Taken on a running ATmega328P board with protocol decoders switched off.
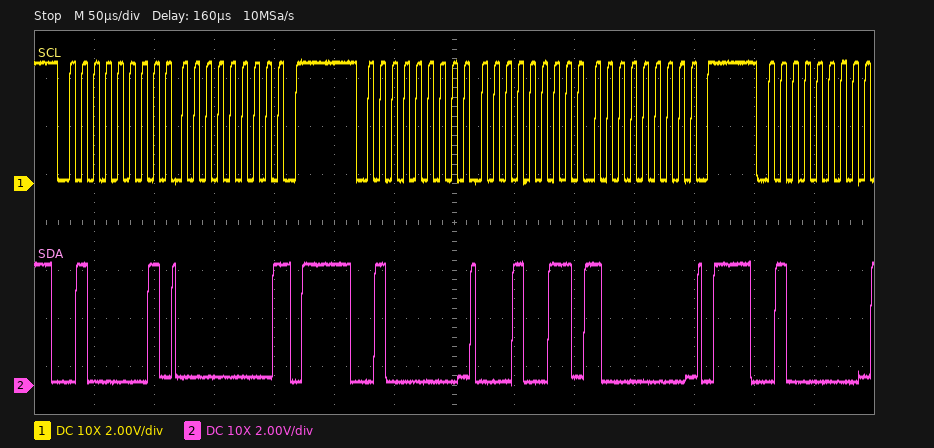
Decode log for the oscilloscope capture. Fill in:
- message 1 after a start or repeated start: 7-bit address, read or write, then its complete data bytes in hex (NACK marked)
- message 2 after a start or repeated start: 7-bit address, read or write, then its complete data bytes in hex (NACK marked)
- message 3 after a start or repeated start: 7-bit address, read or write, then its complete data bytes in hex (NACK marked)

0x20 read: 00 NACK
0x20 write: 13 80
0x20 write
